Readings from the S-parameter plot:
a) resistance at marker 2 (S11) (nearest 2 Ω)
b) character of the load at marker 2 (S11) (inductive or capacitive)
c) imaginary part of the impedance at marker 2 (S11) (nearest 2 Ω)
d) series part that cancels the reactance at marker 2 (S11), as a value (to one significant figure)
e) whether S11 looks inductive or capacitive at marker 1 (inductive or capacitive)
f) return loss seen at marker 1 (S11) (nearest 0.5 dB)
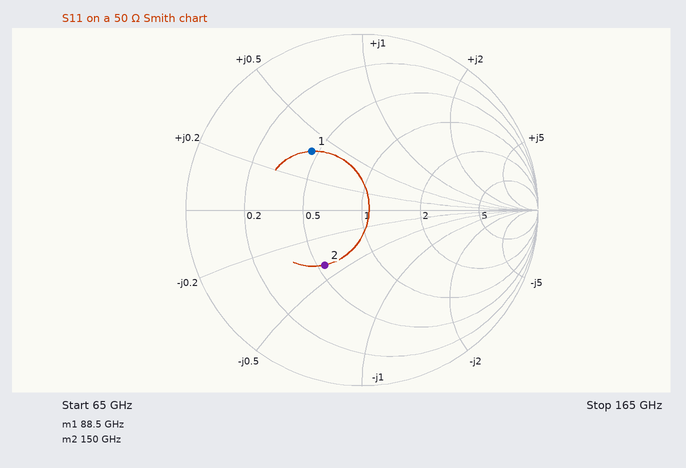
28 Ω
capacitive
-20 Ω
20 pH
inductive
7.0 dB
